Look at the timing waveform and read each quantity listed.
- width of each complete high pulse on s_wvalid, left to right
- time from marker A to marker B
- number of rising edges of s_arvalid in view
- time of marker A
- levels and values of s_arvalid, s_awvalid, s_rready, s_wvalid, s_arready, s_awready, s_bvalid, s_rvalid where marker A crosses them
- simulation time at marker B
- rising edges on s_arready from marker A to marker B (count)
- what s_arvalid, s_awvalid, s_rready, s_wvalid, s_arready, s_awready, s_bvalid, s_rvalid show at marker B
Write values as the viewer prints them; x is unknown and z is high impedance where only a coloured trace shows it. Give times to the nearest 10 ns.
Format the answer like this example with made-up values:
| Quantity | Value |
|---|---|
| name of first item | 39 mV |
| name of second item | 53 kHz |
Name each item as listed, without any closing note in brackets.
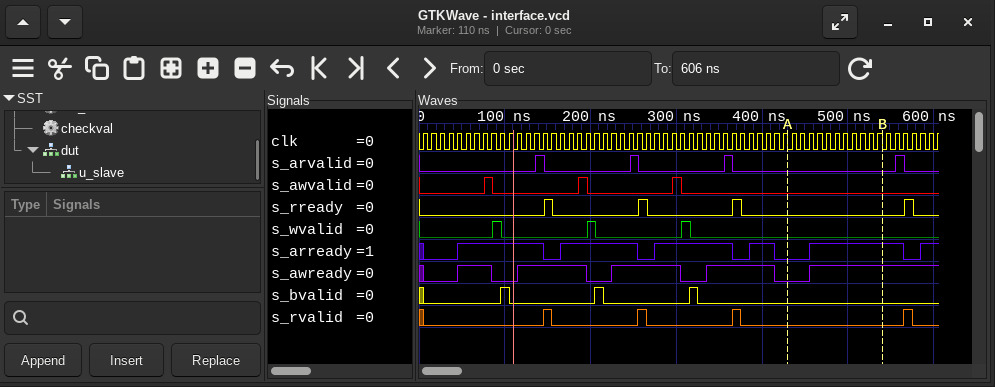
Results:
| Quantity | Value |
|---|---|
| width of each complete high pulse on s_wvalid, left to right | 10 ns, 10 ns, 10 ns |
| time from marker A to marker B | 110 ns |
| number of rising edges of s_arvalid in view | 4 |
| time of marker A | 430 ns |
| levels and values of s_arvalid, s_awvalid, s_rready, s_wvalid, s_arready, s_awready, s_bvalid, s_rvalid where marker A crosses them | s_arvalid=0, s_awvalid=0, s_rready=0, s_wvalid=0, s_arready=0, s_awready=0, s_bvalid=0, s_rvalid=0 |
| simulation time at marker B | 540 ns |
| rising edges on s_arready from marker A to marker B | 1 |
| what s_arvalid, s_awvalid, s_rready, s_wvalid, s_arready, s_awready, s_bvalid, s_rvalid show at marker B | s_arvalid=0, s_awvalid=0, s_rready=0, s_wvalid=0, s_arready=1, s_awready=1, s_bvalid=0, s_rvalid=0 |
